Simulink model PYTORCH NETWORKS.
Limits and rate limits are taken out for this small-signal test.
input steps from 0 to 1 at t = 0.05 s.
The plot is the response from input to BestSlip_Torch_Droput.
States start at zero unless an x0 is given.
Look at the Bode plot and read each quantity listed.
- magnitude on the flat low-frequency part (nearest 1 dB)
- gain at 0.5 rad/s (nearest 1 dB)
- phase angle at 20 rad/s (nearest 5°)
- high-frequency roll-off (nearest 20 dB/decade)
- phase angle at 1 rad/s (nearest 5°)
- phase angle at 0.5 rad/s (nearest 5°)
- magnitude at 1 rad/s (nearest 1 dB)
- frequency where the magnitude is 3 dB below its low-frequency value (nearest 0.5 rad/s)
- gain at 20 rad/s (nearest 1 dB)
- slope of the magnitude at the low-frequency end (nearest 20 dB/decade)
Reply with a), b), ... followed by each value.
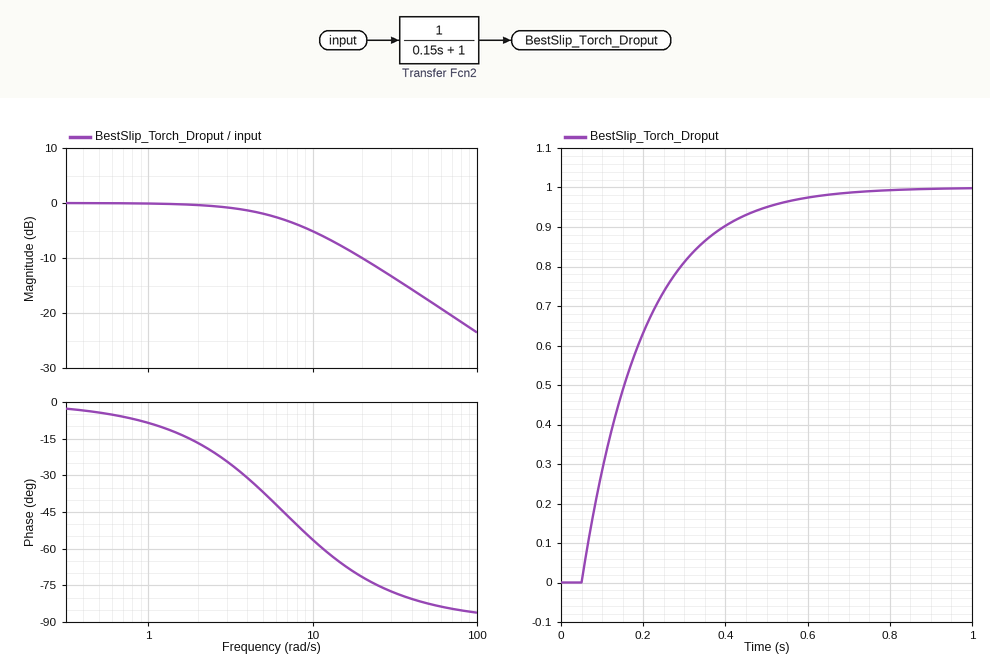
a) 0 dB
b) 0 dB
c) -70°
d) -20 dB/decade
e) -10°
f) -5°
g) 0 dB
h) 6.5 rad/s
i) -10 dB
j) 0 dB/decade
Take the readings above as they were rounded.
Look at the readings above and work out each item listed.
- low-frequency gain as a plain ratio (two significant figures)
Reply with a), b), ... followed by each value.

a) 1.0
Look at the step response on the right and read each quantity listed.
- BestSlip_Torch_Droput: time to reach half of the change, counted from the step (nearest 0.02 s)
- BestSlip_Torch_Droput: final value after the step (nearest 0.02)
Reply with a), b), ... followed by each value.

a) 0.10 s
b) 1.00
